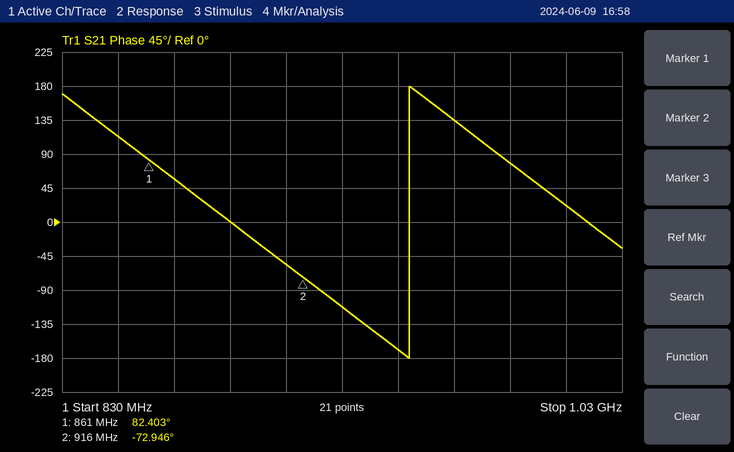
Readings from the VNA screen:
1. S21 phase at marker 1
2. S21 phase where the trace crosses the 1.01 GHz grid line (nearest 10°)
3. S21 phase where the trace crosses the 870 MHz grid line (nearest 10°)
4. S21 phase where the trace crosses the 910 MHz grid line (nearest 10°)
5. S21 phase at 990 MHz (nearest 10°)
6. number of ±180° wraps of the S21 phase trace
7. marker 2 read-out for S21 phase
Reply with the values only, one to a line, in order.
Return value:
82.403°
20°
60°
-60°
80°
1
-72.946°
